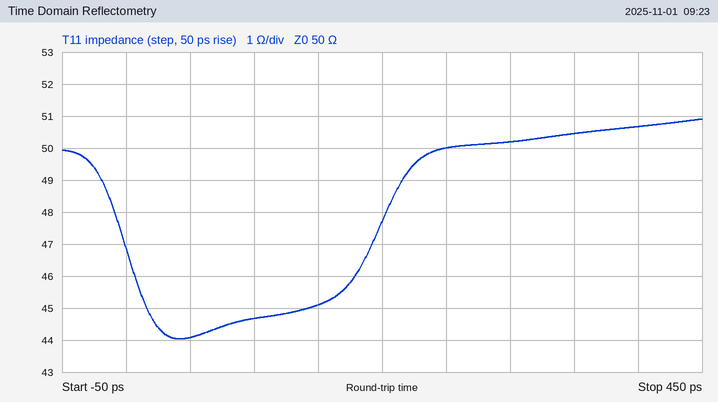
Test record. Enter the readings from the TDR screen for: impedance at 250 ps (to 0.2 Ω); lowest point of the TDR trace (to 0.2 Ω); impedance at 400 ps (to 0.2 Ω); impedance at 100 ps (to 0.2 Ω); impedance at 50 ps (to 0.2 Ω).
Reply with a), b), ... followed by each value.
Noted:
a) 50.0 Ω
b) 44.0 Ω
c) 50.6 Ω
d) 44.6 Ω
e) 44.0 Ω
